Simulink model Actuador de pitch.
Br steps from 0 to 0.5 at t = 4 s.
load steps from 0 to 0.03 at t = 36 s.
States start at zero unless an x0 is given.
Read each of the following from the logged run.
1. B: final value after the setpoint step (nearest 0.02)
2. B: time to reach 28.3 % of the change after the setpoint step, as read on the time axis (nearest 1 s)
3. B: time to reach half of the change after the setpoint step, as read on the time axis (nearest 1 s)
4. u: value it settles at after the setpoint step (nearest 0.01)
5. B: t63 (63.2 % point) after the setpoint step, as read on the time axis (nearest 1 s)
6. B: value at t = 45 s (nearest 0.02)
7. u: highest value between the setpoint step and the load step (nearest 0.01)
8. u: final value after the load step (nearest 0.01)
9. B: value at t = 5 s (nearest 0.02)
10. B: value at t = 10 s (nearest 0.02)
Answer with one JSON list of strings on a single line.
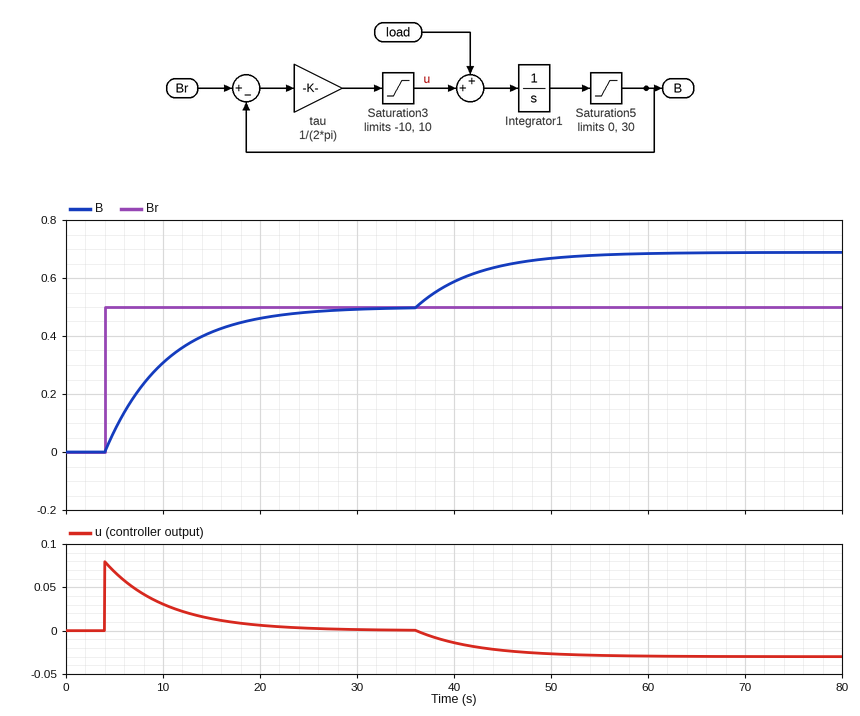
["0.50", "6 s", "8 s", "0.00", "10 s", "0.64", "0.08", "-0.03", "0.08", "0.30"]
